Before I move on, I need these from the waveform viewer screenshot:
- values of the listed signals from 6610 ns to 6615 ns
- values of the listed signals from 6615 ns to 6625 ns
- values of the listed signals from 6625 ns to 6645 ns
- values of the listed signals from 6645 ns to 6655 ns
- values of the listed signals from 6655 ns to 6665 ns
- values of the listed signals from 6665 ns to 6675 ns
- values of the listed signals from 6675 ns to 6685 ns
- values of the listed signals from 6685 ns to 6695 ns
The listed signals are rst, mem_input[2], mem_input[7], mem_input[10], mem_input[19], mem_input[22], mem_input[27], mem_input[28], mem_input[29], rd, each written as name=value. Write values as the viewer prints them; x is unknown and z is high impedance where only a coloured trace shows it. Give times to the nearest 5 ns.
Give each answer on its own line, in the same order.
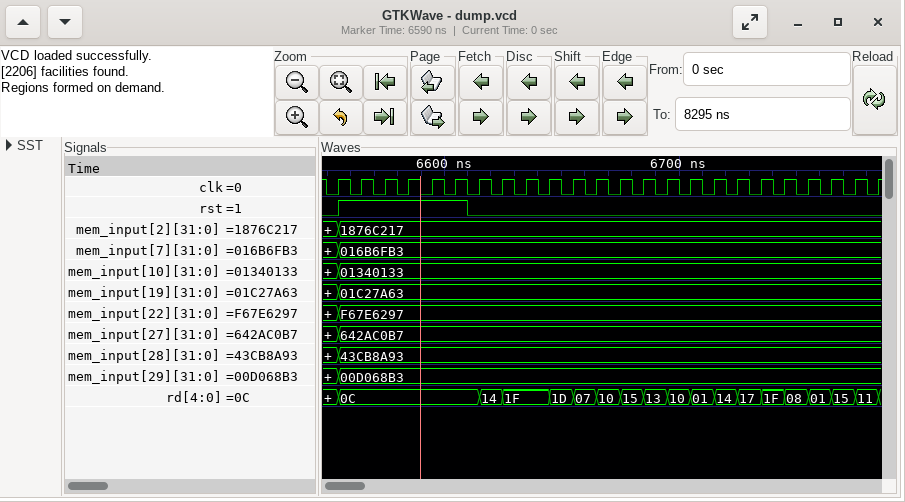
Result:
rst=0, mem_input[2]=1876C217, mem_input[7]=016B6FB3, mem_input[10]=01340133, mem_input[19]=01C27A63, mem_input[22]=F67E6297, mem_input[27]=642AC0B7, mem_input[28]=43CB8A93, mem_input[29]=00D068B3, rd=0C
rst=0, mem_input[2]=1876C217, mem_input[7]=016B6FB3, mem_input[10]=01340133, mem_input[19]=01C27A63, mem_input[22]=F67E6297, mem_input[27]=642AC0B7, mem_input[28]=43CB8A93, mem_input[29]=00D068B3, rd=14
rst=0, mem_input[2]=1876C217, mem_input[7]=016B6FB3, mem_input[10]=01340133, mem_input[19]=01C27A63, mem_input[22]=F67E6297, mem_input[27]=642AC0B7, mem_input[28]=43CB8A93, mem_input[29]=00D068B3, rd=1F
rst=0, mem_input[2]=1876C217, mem_input[7]=016B6FB3, mem_input[10]=01340133, mem_input[19]=01C27A63, mem_input[22]=F67E6297, mem_input[27]=642AC0B7, mem_input[28]=43CB8A93, mem_input[29]=00D068B3, rd=1D
rst=0, mem_input[2]=1876C217, mem_input[7]=016B6FB3, mem_input[10]=01340133, mem_input[19]=01C27A63, mem_input[22]=F67E6297, mem_input[27]=642AC0B7, mem_input[28]=43CB8A93, mem_input[29]=00D068B3, rd=07
rst=0, mem_input[2]=1876C217, mem_input[7]=016B6FB3, mem_input[10]=01340133, mem_input[19]=01C27A63, mem_input[22]=F67E6297, mem_input[27]=642AC0B7, mem_input[28]=43CB8A93, mem_input[29]=00D068B3, rd=10
rst=0, mem_input[2]=1876C217, mem_input[7]=016B6FB3, mem_input[10]=01340133, mem_input[19]=01C27A63, mem_input[22]=F67E6297, mem_input[27]=642AC0B7, mem_input[28]=43CB8A93, mem_input[29]=00D068B3, rd=15
rst=0, mem_input[2]=1876C217, mem_input[7]=016B6FB3, mem_input[10]=01340133, mem_input[19]=01C27A63, mem_input[22]=F67E6297, mem_input[27]=642AC0B7, mem_input[28]=43CB8A93, mem_input[29]=00D068B3, rd=13
